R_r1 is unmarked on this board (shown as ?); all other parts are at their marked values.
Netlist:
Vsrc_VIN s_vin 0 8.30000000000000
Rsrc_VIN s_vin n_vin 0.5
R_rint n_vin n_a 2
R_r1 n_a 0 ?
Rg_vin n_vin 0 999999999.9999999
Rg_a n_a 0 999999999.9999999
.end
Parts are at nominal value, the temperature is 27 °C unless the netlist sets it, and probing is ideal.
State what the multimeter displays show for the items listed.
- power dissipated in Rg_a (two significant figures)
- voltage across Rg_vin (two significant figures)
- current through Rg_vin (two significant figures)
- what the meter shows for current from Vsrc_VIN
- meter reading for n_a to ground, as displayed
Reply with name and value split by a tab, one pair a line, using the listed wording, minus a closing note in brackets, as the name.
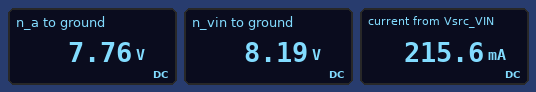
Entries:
power dissipated in Rg_a	60 nW
voltage across Rg_vin	8.2 V
current through Rg_vin	8.2 nA
what the meter shows for current from Vsrc_VIN	215.6 mA
meter reading for n_a to ground, as displayed	7.76 V
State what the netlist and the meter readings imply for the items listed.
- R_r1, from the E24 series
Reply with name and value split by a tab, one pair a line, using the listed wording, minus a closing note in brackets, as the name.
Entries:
R_r1, from the E24 series	36 Ω
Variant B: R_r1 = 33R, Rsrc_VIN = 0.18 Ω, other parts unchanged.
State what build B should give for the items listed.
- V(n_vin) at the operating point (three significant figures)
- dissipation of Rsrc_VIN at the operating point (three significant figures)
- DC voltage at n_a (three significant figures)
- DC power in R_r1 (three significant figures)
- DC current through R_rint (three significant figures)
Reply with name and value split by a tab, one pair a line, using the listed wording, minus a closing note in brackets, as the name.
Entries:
V(n_vin) at the operating point	8.26 V
dissipation of Rsrc_VIN at the operating point	10.0 mW
DC voltage at n_a	7.79 V
DC power in R_r1	1.84 W
DC current through R_rint	236 mA
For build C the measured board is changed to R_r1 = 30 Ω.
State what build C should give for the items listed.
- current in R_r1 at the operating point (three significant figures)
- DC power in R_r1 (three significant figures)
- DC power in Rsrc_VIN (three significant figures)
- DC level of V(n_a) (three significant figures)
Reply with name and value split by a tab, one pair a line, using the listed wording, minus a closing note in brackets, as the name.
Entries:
current in R_r1 at the operating point	255 mA
DC power in R_r1	1.96 W
DC power in Rsrc_VIN	32.6 mW
DC level of V(n_a)	7.66 V
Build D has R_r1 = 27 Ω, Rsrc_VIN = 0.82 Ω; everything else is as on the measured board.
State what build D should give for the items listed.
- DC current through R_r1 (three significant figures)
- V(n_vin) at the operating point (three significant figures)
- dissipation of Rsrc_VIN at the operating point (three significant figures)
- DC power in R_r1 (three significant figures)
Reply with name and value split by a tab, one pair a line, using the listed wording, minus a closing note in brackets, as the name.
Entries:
DC current through R_r1	278 mA
V(n_vin) at the operating point	8.07 V
dissipation of Rsrc_VIN at the operating point	63.5 mW
DC power in R_r1	2.09 W
